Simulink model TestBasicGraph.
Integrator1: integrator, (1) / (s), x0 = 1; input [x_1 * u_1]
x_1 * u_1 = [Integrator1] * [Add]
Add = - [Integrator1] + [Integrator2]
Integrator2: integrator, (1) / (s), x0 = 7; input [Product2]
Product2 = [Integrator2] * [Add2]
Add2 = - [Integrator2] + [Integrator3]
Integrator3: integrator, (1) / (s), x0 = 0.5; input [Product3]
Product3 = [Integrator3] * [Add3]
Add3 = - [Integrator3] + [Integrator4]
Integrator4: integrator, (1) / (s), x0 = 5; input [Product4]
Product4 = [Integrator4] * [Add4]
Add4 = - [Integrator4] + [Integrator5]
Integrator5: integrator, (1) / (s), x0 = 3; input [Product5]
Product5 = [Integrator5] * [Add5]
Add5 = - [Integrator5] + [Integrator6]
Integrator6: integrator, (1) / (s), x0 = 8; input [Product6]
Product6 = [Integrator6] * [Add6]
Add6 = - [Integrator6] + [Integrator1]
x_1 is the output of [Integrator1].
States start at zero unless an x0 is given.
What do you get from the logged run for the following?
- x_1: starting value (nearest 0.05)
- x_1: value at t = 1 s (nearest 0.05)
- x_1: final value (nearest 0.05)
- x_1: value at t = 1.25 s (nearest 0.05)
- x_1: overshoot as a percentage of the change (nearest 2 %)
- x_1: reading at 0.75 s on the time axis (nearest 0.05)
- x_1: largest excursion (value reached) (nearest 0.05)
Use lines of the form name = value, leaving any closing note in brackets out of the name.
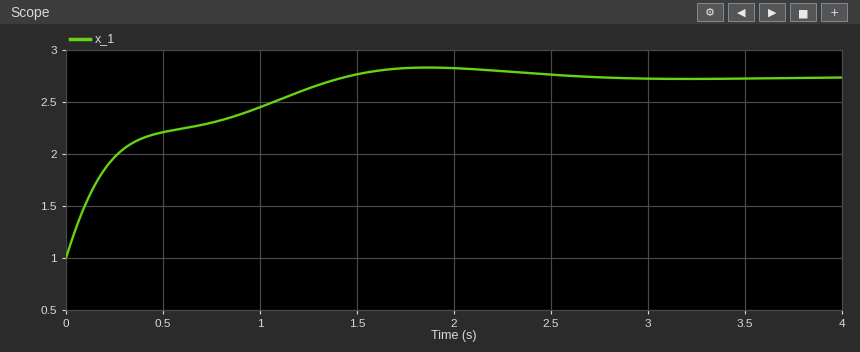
x_1: starting value = 1.00
x_1: value at t = 1 s = 2.45
x_1: final value = 2.75
x_1: value at t = 1.25 s = 2.65
x_1: overshoot as a percentage of the change = 6 %
x_1: reading at 0.75 s on the time axis = 2.30
x_1: largest excursion (value reached) = 2.85
